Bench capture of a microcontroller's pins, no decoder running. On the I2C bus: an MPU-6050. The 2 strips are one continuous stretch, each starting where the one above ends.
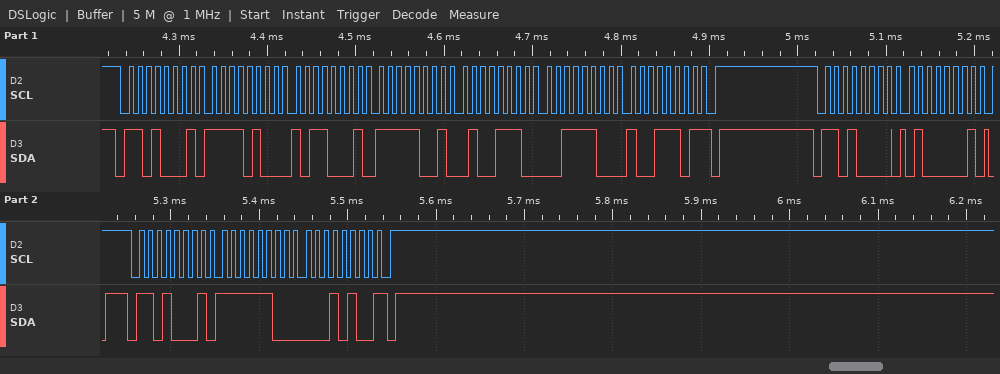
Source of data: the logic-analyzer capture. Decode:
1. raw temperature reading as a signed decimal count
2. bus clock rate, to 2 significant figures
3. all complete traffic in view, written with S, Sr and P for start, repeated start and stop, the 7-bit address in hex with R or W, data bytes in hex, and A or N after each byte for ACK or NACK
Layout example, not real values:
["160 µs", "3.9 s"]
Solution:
["-1004", "100 kHz", "S 68R A F4 A B1 A F9 A 4E A 3C A 9D N P S 68W A 41 A P S 68R A FC A 14 N P"]
